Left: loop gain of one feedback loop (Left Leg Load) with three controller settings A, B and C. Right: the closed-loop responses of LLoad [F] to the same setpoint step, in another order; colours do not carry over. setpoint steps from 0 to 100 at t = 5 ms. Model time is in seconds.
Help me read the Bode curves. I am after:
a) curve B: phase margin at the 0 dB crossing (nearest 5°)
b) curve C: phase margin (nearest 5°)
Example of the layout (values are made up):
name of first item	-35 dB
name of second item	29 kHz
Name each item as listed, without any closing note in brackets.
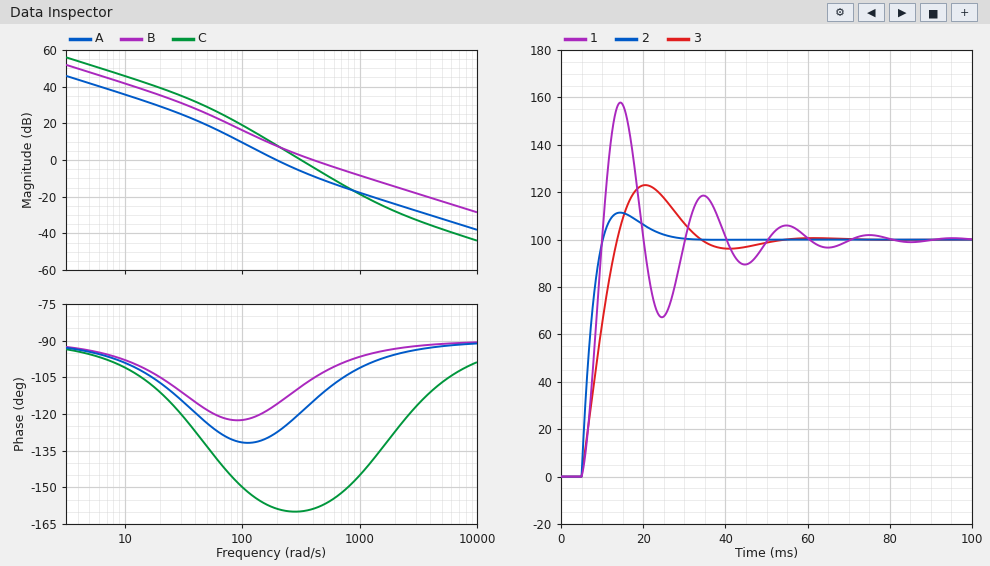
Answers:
curve B: phase margin at the 0 dB crossing	75°
curve C: phase margin	20°
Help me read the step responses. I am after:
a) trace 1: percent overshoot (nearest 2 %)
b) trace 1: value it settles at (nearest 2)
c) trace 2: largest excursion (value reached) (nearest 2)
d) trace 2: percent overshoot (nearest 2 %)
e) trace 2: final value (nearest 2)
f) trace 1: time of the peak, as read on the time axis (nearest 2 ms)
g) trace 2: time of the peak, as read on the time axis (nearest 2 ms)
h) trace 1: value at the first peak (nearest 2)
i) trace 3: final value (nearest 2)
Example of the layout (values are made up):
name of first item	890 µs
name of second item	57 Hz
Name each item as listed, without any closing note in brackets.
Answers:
trace 1: percent overshoot	58 %
trace 1: value it settles at	100
trace 2: largest excursion (value reached)	112
trace 2: percent overshoot	12 %
trace 2: final value	100
trace 1: time of the peak, as read on the time axis	14 ms
trace 2: time of the peak, as read on the time axis	14 ms
trace 1: value at the first peak	158
trace 3: final value	100
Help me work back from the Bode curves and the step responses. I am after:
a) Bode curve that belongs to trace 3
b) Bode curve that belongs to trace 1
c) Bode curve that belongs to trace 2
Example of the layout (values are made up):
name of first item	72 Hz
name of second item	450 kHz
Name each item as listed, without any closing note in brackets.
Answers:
Bode curve that belongs to trace 3	A
Bode curve that belongs to trace 1	C
Bode curve that belongs to trace 2	B
